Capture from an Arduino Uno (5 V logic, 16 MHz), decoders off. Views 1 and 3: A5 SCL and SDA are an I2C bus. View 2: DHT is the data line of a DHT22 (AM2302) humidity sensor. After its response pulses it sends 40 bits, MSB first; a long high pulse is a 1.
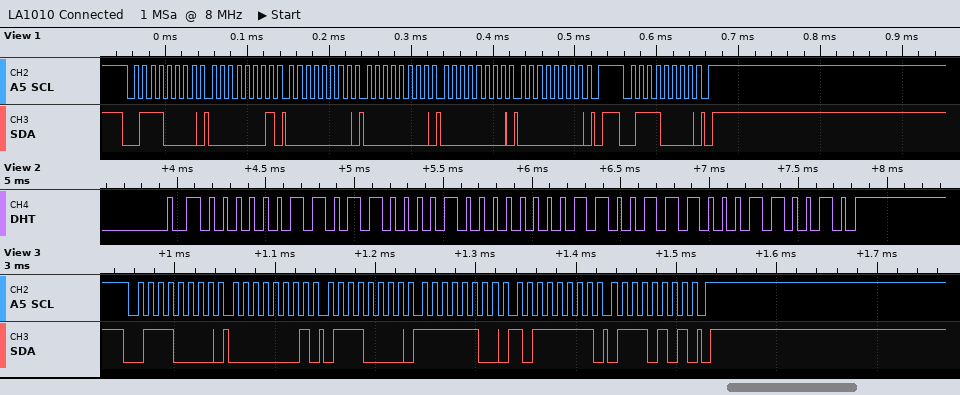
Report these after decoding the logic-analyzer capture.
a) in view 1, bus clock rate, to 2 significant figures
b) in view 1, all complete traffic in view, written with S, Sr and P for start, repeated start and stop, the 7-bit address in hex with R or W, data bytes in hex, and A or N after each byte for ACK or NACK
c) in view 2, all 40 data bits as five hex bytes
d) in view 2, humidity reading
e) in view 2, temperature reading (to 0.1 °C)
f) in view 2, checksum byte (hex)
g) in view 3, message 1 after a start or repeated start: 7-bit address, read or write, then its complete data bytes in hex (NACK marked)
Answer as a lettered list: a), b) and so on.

a) 100 kHz
b) S 38W A 01 A 00 A 00 A 00 A 00 A P S 38W A P
c) 03 61 00 CE 32
d) 86.5 %
e) 20.6 °C
f) 0x32
g) 0x38 write: 01 70 FC BF 75
